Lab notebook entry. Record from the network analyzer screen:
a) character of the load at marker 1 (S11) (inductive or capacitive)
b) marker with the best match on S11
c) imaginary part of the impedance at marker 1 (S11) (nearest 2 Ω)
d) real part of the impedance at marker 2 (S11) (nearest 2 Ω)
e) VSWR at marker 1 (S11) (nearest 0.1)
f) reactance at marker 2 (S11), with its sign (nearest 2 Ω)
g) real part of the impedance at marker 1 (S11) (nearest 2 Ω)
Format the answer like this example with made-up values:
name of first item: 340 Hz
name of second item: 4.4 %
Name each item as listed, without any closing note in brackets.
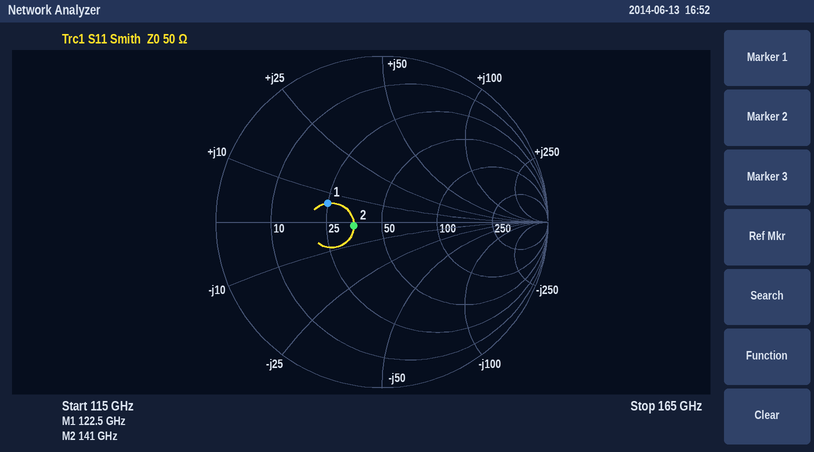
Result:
character of the load at marker 1 (S11): inductive
marker with the best match on S11: marker 2
imaginary part of the impedance at marker 1 (S11): +6 Ω
real part of the impedance at marker 2 (S11): 36 Ω
VSWR at marker 1 (S11): 2.1
reactance at marker 2 (S11), with its sign: -2 Ω
real part of the impedance at marker 1 (S11): 24 Ω
